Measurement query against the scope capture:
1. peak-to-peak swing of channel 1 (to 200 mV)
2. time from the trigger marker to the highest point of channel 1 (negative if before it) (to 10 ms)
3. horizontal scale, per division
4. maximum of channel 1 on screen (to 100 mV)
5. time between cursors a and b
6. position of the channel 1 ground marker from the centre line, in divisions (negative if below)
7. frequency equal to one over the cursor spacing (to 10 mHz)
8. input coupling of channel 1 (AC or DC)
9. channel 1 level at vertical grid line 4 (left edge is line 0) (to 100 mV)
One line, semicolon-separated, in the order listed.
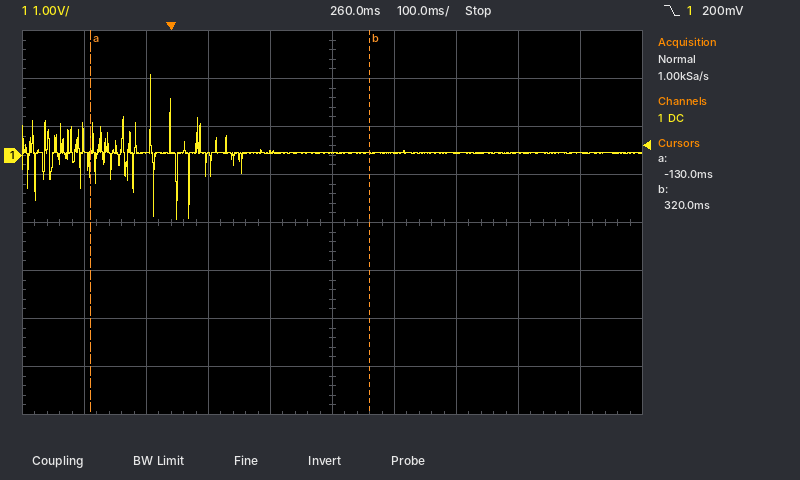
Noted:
3.0 V; -30 ms; 100 ms; 1.7 V; 450 ms; +1.4 div; 2.22 Hz; DC; 100 mV
